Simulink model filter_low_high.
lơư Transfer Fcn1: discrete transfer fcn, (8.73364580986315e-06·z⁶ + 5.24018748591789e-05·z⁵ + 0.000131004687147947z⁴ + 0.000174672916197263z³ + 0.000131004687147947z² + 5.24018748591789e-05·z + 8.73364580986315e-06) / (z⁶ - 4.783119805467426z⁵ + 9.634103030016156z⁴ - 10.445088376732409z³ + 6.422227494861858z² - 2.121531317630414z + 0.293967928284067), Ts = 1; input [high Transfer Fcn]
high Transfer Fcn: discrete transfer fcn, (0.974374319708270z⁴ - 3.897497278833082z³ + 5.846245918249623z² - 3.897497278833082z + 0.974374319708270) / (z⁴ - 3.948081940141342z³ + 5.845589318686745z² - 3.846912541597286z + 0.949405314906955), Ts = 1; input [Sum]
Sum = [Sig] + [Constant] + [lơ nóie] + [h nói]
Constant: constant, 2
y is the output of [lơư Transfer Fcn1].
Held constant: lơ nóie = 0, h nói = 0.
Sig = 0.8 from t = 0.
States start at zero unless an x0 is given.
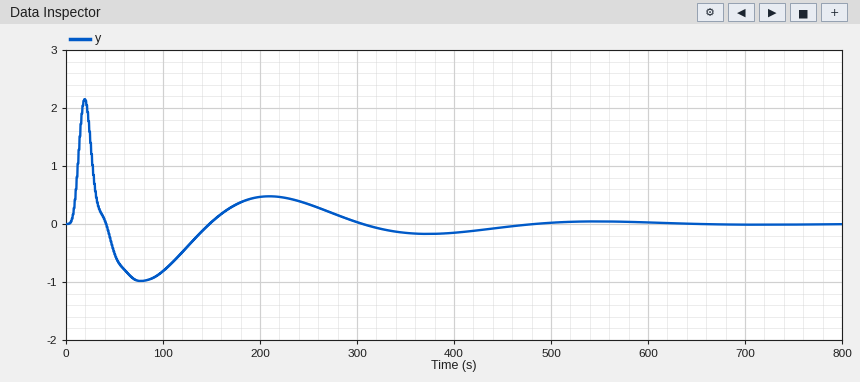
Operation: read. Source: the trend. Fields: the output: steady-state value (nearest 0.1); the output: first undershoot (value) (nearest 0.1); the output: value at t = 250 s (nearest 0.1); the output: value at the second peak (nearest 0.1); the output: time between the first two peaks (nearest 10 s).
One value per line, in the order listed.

0.0
-1.0
0.3
0.5
190 s
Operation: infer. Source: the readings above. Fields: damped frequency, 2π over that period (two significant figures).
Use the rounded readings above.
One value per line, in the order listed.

0.033 rad/s
